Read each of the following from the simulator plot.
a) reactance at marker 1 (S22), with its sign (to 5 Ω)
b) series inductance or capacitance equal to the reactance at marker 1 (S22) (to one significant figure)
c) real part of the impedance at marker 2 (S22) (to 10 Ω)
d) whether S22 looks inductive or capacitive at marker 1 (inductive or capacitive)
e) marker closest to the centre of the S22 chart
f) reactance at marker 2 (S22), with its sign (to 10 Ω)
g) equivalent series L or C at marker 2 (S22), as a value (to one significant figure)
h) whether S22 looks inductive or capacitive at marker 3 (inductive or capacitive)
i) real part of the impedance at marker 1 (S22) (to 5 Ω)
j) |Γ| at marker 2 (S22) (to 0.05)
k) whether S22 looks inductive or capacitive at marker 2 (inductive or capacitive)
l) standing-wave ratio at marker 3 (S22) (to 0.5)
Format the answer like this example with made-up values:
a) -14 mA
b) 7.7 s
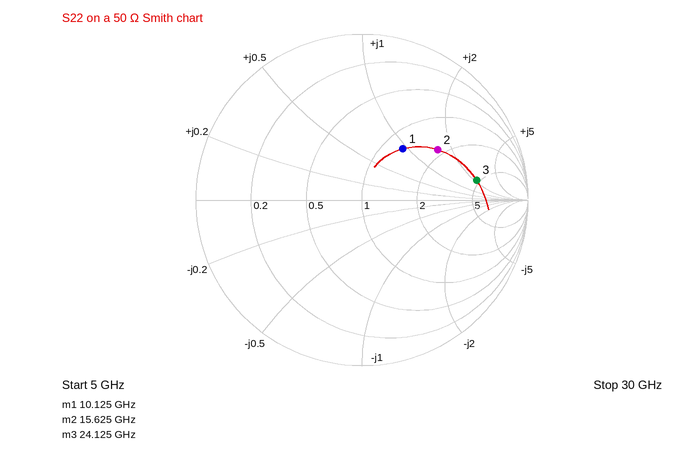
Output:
a) +45 Ω
b) 700 pH
c) 90 Ω
d) inductive
e) marker 1
f) +80 Ω
g) 800 pH
h) inductive
i) 65 Ω
j) 0.55
k) inductive
l) 5.5
